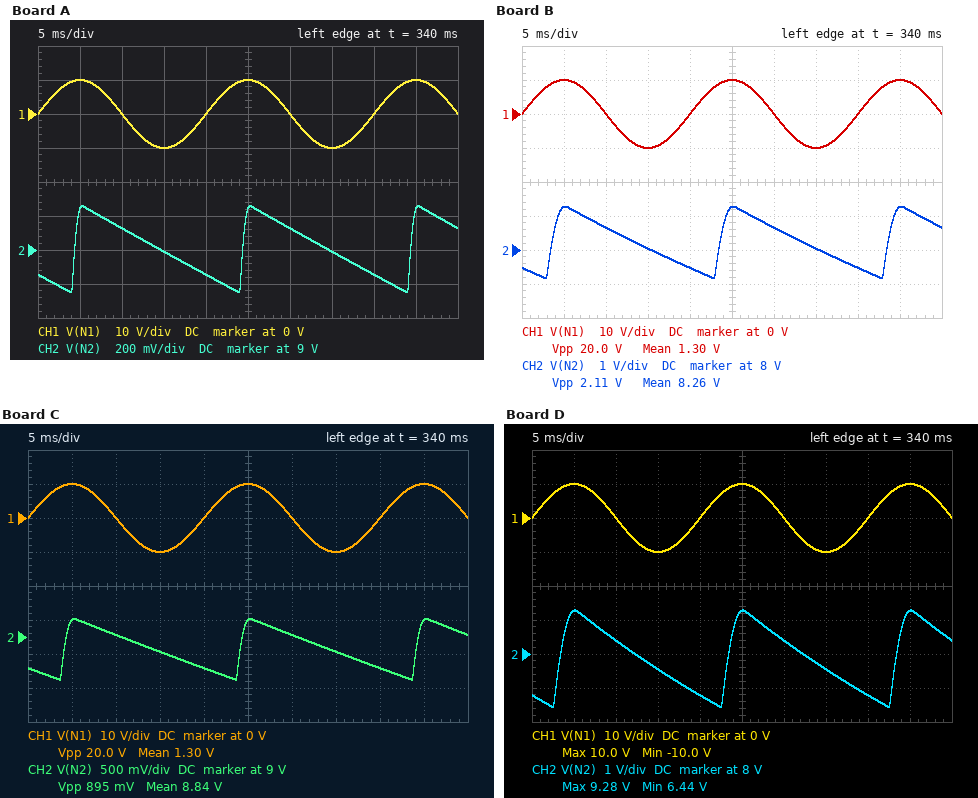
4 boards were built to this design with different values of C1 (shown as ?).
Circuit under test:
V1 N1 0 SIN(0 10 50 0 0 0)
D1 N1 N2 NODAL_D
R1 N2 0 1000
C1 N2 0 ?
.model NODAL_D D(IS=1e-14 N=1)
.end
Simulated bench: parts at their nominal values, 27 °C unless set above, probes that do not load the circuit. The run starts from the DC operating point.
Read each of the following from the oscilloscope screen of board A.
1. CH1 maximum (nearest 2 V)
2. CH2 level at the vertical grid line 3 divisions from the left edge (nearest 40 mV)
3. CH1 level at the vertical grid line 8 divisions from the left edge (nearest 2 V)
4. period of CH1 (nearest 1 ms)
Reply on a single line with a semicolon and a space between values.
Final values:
10 V; 9.00 V; 0 V; 20 ms
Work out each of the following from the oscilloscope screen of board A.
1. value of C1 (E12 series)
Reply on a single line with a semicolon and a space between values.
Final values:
330 µF
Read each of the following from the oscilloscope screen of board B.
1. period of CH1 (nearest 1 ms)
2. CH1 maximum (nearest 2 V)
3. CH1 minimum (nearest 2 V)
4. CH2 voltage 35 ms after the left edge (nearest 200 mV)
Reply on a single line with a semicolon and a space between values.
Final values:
20 ms; 10 V; -10 V; 8.0 V
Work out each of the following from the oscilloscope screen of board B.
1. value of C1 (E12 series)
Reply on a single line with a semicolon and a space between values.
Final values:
68 µF
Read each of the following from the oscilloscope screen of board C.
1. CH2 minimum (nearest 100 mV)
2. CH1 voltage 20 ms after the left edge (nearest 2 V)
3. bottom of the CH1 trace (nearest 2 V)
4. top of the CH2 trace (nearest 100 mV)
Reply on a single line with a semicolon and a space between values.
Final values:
8.4 V; 0 V; -10 V; 9.3 V
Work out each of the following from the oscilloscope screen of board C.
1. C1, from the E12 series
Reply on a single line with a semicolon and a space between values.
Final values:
180 µF
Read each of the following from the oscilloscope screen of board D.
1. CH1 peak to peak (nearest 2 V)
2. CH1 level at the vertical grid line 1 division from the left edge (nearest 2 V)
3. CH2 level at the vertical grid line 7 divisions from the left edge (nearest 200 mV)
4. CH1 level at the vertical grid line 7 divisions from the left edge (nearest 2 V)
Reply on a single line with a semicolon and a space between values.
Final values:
20 V; 10 V; 7.6 V; -10 V
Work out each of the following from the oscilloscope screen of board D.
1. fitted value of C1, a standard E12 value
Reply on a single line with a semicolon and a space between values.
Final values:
47 µF
